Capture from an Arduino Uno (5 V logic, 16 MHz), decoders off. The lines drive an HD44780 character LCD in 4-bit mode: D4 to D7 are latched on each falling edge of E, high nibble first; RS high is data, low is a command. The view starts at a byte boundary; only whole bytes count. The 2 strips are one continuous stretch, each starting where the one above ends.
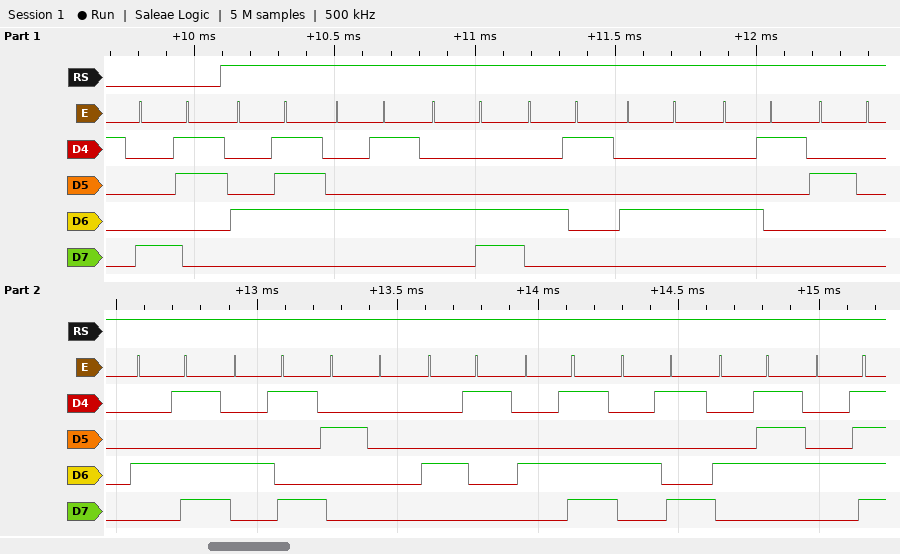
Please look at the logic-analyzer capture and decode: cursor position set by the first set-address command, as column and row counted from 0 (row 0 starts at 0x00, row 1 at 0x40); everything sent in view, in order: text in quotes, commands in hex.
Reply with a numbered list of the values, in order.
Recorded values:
1. column 3, row 0
2. 0x83 "GELADA MI AMIGO"
